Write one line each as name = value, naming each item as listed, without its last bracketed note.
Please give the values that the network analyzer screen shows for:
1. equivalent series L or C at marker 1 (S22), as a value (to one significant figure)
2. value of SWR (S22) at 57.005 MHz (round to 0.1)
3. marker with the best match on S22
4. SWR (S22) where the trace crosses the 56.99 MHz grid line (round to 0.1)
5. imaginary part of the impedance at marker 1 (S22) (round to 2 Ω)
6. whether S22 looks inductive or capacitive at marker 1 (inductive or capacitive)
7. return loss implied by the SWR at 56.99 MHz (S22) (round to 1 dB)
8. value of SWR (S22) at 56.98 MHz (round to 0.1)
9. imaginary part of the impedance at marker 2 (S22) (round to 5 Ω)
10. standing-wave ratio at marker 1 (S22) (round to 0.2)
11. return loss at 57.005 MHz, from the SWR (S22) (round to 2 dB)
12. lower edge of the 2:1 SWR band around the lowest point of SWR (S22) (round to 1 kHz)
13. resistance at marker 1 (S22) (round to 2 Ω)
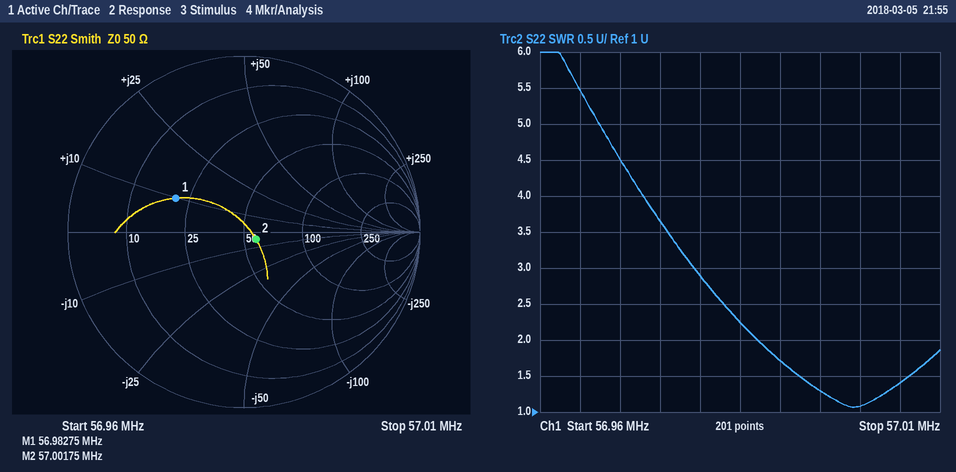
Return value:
equivalent series L or C at marker 1 (S22), as a value = 30 nH
value of SWR (S22) at 57.005 MHz = 1.4
marker with the best match on S22 = marker 2
SWR (S22) where the trace crosses the 56.99 MHz grid line = 1.7
imaginary part of the impedance at marker 1 (S22) = +10 Ω
whether S22 looks inductive or capacitive at marker 1 = inductive
return loss implied by the SWR at 56.99 MHz (S22) = 12 dB
value of SWR (S22) at 56.98 MHz = 2.9
imaginary part of the impedance at marker 2 (S22) = -5 Ω
standing-wave ratio at marker 1 (S22) = 2.6
return loss at 57.005 MHz, from the SWR (S22) = 16 dB
lower edge of the 2:1 SWR band around the lowest point of SWR (S22) = 56.987 MHz
resistance at marker 1 (S22) = 20 Ω
